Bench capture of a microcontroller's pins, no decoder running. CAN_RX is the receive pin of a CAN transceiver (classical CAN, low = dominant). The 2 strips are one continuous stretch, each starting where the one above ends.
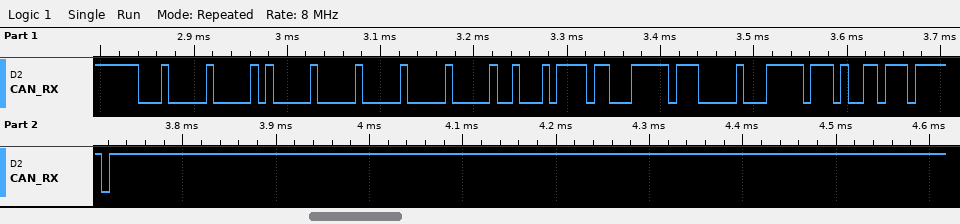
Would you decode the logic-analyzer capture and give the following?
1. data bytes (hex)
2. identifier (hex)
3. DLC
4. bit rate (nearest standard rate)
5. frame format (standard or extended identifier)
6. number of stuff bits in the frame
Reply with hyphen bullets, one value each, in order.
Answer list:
- 00 00 00 8B D8 FF 00 FF
- 0x100
- 8
- 125 kbit/s
- standard
- 10
